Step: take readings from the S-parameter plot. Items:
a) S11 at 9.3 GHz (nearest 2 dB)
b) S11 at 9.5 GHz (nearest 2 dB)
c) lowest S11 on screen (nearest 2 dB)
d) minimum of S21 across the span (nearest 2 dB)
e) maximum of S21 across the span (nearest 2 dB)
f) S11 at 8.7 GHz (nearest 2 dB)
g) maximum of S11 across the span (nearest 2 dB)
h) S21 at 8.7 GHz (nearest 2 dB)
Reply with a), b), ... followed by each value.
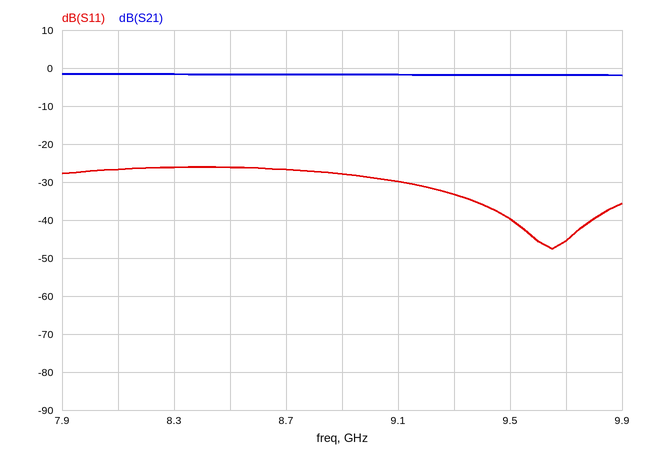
a) -34 dB
b) -40 dB
c) -48 dB
d) -2 dB
e) -2 dB
f) -26 dB
g) -26 dB
h) -2 dB
